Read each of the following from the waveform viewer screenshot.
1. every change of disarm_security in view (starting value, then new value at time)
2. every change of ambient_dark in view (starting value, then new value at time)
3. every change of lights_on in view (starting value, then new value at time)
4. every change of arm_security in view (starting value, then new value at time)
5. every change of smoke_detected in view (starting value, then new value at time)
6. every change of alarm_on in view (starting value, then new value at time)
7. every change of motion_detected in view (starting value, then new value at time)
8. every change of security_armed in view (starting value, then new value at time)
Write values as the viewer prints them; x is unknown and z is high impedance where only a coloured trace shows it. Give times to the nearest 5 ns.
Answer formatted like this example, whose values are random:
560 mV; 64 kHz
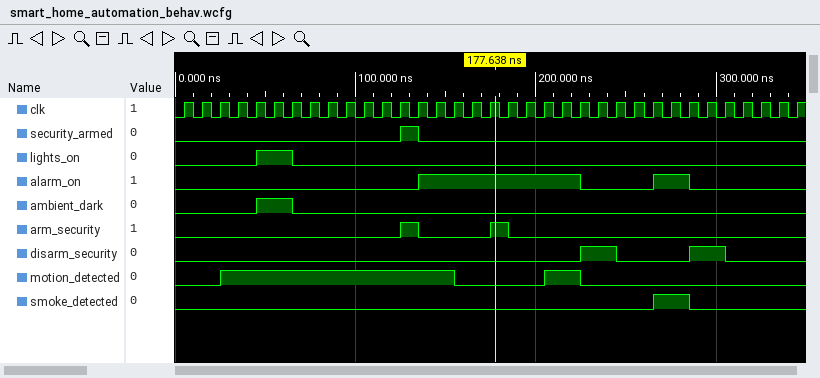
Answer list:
0, 1 at 225 ns, 0 at 245 ns, 1 at 285 ns, 0 at 305 ns; 0, 1 at 45 ns, 0 at 65 ns; 0, 1 at 45 ns, 0 at 65 ns; 0, 1 at 125 ns, 0 at 135 ns, 1 at 175 ns, 0 at 185 ns; 0, 1 at 265 ns, 0 at 285 ns; 0, 1 at 135 ns, 0 at 225 ns, 1 at 265 ns, 0 at 285 ns; 0, 1 at 25 ns, 0 at 155 ns, 1 at 205 ns, 0 at 225 ns; 0, 1 at 125 ns, 0 at 135 ns
